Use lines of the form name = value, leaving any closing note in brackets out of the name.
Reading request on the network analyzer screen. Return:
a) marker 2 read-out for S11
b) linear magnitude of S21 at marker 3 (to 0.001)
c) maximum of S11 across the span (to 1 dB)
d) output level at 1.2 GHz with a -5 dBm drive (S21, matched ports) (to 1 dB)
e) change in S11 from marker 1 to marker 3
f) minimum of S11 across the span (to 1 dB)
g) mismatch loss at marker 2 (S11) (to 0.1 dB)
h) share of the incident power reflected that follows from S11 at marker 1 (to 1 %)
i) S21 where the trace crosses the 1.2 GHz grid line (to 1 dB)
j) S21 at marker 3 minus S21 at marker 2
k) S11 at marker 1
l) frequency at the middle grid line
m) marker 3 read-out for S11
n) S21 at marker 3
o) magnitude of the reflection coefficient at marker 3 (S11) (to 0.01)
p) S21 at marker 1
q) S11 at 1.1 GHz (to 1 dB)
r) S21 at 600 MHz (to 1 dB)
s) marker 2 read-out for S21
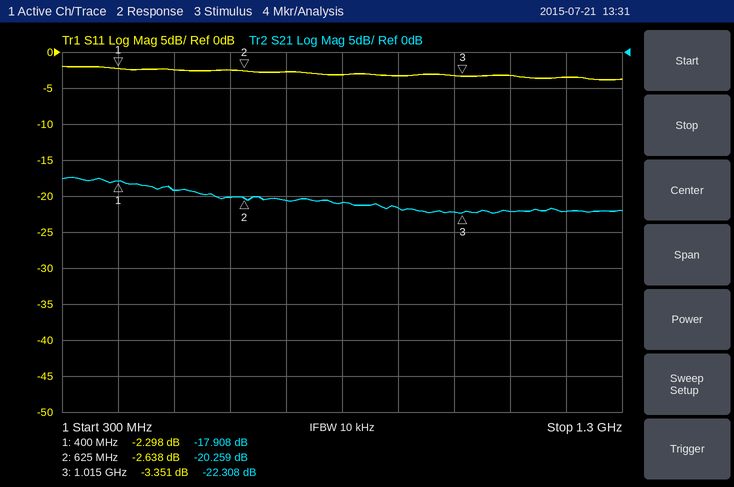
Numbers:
marker 2 read-out for S11 = -2.638 dB
linear magnitude of S21 at marker 3 = 0.077
maximum of S11 across the span = -2 dB
output level at 1.2 GHz with a -5 dBm drive (S21, matched ports) = -27 dBm
change in S11 from marker 1 to marker 3 = -1.053 dB
minimum of S11 across the span = -4 dB
mismatch loss at marker 2 (S11) = 3.4 dB
share of the incident power reflected that follows from S11 at marker 1 = 59 %
S21 where the trace crosses the 1.2 GHz grid line = -22 dB
S21 at marker 3 minus S21 at marker 2 = -2.049 dB
S11 at marker 1 = -2.298 dB
frequency at the middle grid line = 800 MHz
marker 3 read-out for S11 = -3.351 dB
S21 at marker 3 = -22.308 dB
magnitude of the reflection coefficient at marker 3 (S11) = 0.68
S21 at marker 1 = -17.908 dB
S11 at 1.1 GHz = -3 dB
S21 at 600 MHz = -20 dB
marker 2 read-out for S21 = -20.259 dB
